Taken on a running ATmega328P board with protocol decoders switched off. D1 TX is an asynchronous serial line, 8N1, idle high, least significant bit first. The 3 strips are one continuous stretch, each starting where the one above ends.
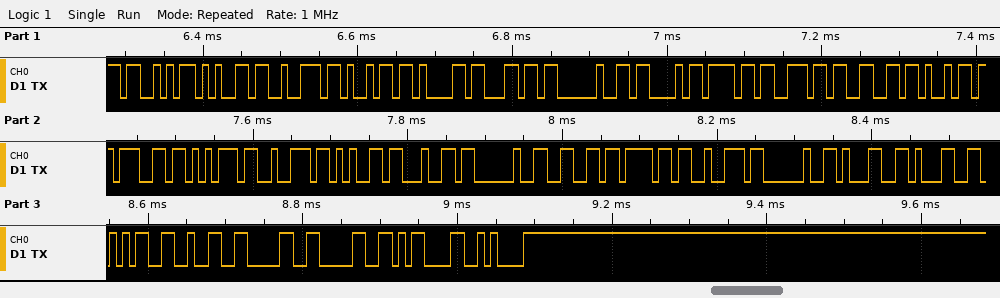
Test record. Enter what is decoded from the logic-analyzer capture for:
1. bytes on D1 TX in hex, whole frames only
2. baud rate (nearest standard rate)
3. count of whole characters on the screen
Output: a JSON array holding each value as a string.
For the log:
["53 65 72 69 61 6C 20 43 6F 6E 66 69 67 75 72 65 64 20 66 6F 72 20 31 31 35 32 30 30 0D 0A", "115200 baud", "30"]
